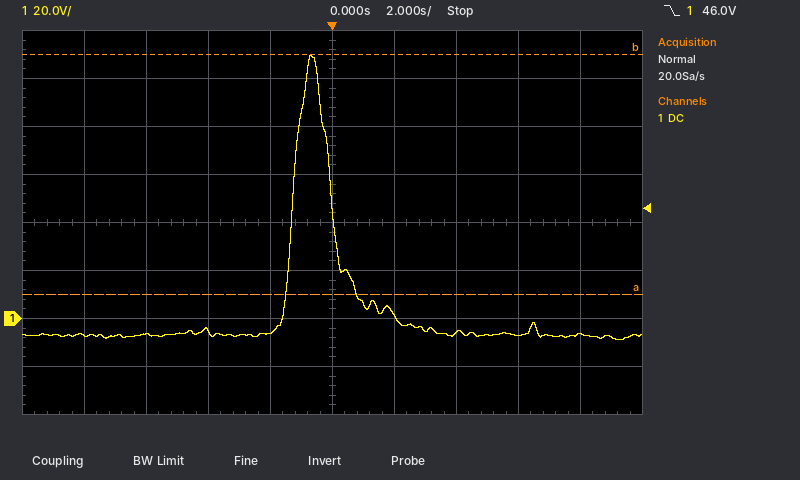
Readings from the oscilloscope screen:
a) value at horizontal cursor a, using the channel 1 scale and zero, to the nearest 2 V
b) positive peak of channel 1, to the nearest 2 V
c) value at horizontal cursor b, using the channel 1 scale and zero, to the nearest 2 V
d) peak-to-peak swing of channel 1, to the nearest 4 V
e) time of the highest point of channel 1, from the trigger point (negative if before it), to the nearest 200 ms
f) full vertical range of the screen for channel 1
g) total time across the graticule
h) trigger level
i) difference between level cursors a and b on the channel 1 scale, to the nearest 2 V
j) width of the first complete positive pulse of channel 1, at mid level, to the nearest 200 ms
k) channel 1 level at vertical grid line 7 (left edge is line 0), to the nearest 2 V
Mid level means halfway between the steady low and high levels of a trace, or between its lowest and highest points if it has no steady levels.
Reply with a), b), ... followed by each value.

a) 10 V
b) 110 V
c) 110 V
d) 120 V
e) -600 ms
f) 160 V
g) 20 s
h) 46.0 V
i) 100 V
j) 1.2 s
k) -6 V
